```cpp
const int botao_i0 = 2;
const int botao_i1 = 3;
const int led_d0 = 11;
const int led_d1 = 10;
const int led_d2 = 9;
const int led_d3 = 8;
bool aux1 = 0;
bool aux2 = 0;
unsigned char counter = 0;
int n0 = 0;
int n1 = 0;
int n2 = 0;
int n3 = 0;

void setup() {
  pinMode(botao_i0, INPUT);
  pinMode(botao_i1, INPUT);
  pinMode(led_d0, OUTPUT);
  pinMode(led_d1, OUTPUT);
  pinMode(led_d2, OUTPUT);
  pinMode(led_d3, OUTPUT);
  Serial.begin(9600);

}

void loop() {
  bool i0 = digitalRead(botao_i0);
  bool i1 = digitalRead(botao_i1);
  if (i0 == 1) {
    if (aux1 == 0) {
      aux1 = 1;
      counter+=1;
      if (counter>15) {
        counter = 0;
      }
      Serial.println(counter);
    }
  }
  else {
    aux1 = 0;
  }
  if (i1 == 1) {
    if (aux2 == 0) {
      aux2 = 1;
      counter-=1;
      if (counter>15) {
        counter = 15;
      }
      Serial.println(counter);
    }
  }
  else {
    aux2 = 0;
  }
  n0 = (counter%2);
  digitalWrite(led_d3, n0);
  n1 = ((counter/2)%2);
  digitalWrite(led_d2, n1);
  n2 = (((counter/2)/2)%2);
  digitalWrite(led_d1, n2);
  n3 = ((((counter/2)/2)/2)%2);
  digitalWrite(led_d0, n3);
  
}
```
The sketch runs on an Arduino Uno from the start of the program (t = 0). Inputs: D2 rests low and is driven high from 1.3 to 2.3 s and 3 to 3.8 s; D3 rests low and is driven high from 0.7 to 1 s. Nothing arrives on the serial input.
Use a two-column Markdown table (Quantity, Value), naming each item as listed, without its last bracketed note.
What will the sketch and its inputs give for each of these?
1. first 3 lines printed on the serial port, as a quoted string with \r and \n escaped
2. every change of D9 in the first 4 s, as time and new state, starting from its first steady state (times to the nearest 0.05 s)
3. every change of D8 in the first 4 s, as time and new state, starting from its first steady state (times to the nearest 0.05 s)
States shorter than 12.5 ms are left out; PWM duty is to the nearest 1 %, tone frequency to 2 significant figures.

| Quantity | Value |
|---|---|
| first 3 lines printed on the serial port, as a quoted string with \r and \n escaped | "15\r\n0\r\n1\r\n" |
| every change of D9 in the first 4 s, as time and new state, starting from its first steady state | 0 s low; 0.7 s high; 1.3 s low |
| every change of D8 in the first 4 s, as time and new state, starting from its first steady state | 0 s low; 0.7 s high; 1.3 s low; 3 s high |
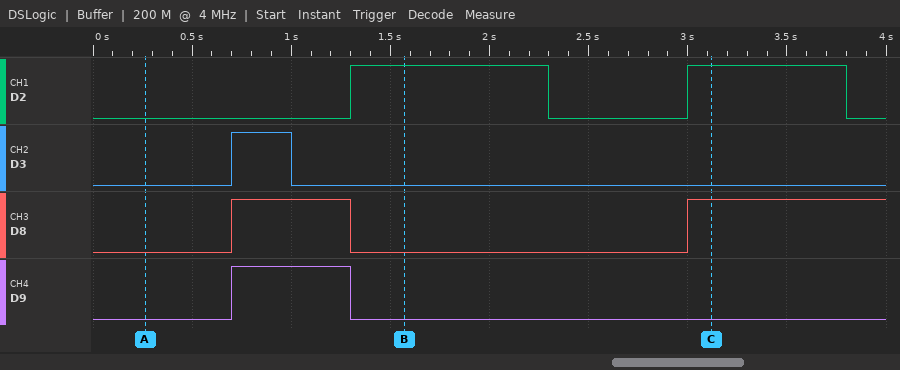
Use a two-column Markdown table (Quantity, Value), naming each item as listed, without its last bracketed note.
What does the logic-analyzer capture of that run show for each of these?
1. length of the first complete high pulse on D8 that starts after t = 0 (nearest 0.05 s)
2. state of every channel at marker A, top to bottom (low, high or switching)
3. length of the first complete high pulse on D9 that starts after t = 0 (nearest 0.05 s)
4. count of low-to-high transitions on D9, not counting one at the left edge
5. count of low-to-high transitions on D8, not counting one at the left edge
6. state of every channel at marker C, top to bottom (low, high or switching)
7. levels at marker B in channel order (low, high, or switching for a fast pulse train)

| Quantity | Value |
|---|---|
| length of the first complete high pulse on D8 that starts after t = 0 | 0.60 s |
| state of every channel at marker A, top to bottom | D2 low, D3 low, D8 low, D9 low |
| length of the first complete high pulse on D9 that starts after t = 0 | 0.60 s |
| count of low-to-high transitions on D9, not counting one at the left edge | 1 |
| count of low-to-high transitions on D8, not counting one at the left edge | 2 |
| state of every channel at marker C, top to bottom | D2 high, D3 low, D8 high, D9 low |
| levels at marker B in channel order | D2 high, D3 low, D8 low, D9 low |
